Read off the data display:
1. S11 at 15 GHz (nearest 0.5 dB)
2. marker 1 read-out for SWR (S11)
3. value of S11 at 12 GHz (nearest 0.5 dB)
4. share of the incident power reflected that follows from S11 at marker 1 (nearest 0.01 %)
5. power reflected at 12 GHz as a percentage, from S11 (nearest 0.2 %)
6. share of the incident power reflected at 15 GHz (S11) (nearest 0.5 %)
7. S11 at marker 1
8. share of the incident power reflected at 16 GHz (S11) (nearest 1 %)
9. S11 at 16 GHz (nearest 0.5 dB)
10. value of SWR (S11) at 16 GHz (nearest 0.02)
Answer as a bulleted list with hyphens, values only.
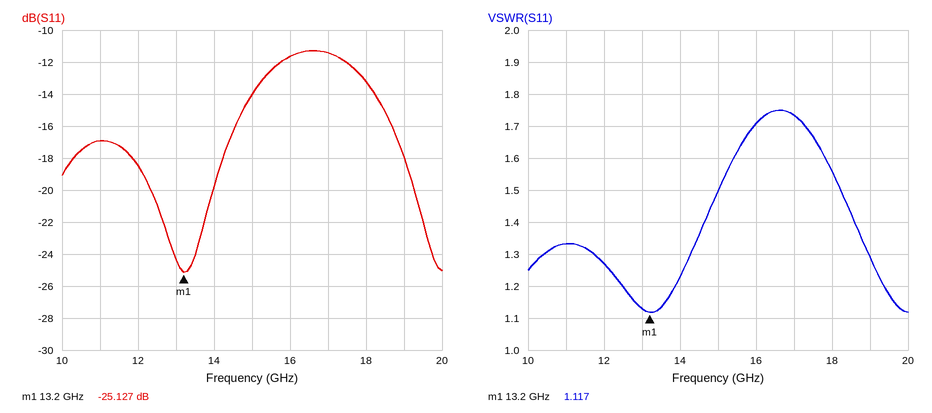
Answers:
- -14.0 dB
- 1.117
- -18.5 dB
- 0.31 %
- 1.4 %
- 4.0 %
- -25.127 dB
- 7 %
- -11.5 dB
- 1.70
